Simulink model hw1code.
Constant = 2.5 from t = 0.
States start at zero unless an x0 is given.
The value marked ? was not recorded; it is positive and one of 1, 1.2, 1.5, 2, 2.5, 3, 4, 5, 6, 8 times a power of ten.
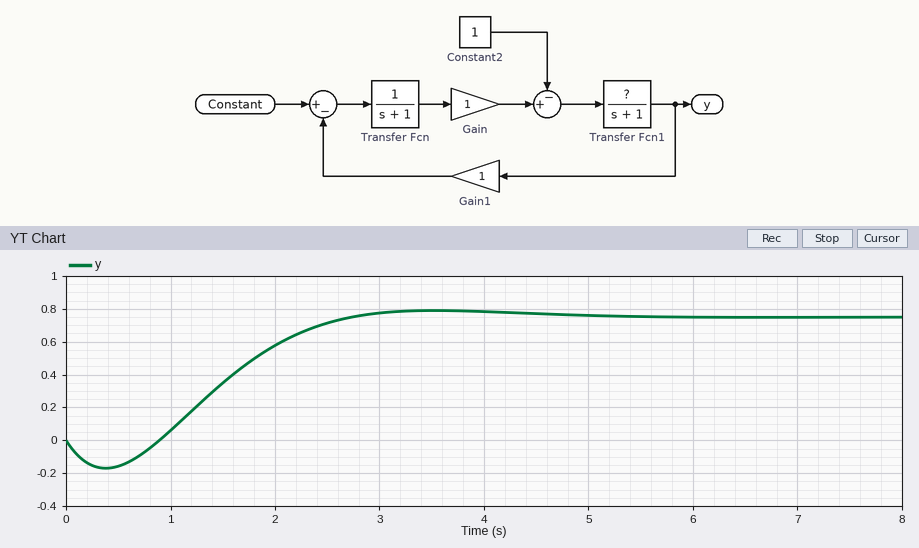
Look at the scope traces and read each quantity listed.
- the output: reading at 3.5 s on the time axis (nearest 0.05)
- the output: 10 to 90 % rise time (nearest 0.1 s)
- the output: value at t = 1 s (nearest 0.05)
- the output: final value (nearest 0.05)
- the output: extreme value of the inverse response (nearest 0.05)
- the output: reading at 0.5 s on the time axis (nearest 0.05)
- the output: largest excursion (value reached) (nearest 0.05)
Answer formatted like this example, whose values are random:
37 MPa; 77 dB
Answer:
0.80; 1.3 s; 0.05; 0.75; -0.15; -0.15; 0.80
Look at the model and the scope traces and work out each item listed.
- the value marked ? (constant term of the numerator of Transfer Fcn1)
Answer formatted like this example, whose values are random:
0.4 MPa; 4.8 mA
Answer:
1
